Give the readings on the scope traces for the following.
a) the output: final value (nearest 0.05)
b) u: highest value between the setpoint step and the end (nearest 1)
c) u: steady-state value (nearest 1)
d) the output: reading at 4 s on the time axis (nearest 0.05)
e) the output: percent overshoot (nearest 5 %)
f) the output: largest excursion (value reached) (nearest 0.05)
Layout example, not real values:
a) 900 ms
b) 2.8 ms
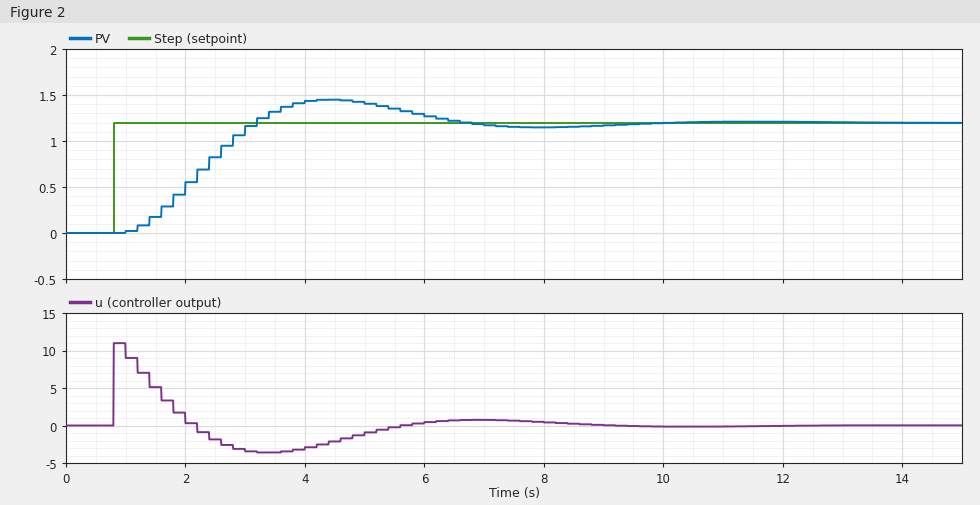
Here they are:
a) 1.20
b) 11
c) 0
d) 1.45
e) 20 %
f) 1.45
